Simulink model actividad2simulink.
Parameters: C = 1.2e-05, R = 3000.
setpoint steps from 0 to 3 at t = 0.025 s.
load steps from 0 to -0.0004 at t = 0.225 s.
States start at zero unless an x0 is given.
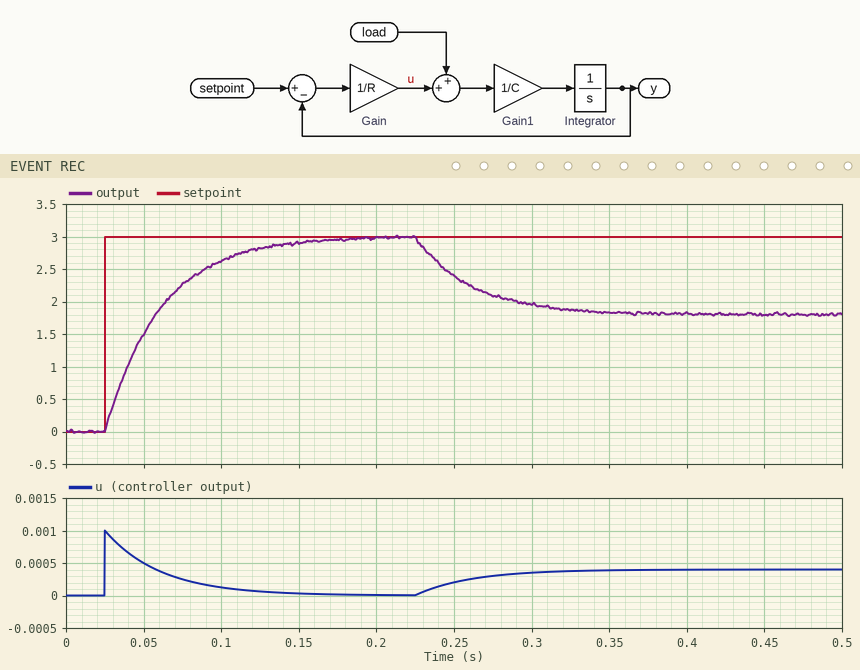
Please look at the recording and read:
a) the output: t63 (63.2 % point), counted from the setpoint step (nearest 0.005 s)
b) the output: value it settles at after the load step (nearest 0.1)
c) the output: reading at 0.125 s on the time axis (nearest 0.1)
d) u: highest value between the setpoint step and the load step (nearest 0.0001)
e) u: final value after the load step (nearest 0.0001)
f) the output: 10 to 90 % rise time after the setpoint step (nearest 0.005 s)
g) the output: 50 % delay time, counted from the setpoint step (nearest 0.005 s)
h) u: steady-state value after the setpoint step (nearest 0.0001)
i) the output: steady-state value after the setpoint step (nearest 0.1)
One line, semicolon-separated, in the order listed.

0.035 s; 1.8; 2.8; 0.0010; 0.0004; 0.080 s; 0.025 s; 0.0000; 3.0
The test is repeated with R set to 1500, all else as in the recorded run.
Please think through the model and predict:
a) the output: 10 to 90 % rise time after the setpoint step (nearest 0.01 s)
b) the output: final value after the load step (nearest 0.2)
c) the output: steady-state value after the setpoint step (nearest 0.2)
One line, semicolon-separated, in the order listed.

0.04 s; 2.4; 3.0
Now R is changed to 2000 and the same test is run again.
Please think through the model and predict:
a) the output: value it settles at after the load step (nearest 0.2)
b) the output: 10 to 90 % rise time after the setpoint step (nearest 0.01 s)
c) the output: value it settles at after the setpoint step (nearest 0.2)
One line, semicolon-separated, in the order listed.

2.2; 0.05 s; 3.0
